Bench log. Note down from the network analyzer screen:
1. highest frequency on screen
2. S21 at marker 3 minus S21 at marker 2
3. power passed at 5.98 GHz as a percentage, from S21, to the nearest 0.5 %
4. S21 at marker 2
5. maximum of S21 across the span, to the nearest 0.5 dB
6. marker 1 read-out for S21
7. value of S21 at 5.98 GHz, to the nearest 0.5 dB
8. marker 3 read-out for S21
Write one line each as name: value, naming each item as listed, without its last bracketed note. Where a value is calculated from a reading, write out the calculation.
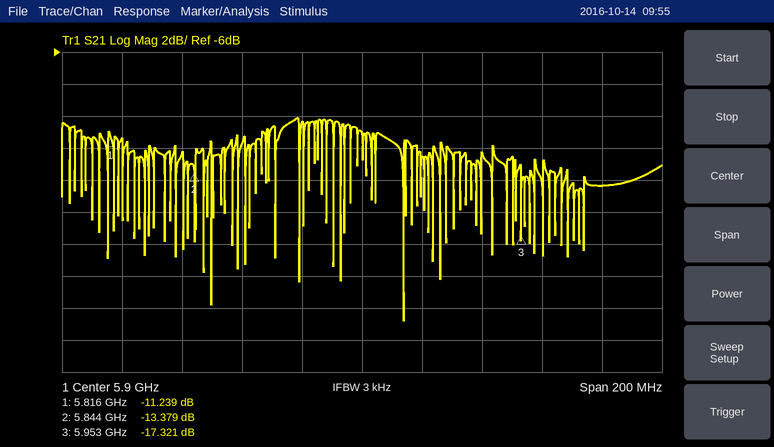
highest frequency on screen: 6 GHz
S21 at marker 3 minus S21 at marker 2: -17.321 − (-13.379) = -3.942 dB
power passed at 5.98 GHz as a percentage, from S21, to the nearest 0.5 %: 10^(-14.5/10) ≈ 3.5 %
S21 at marker 2: -13.379 dB
maximum of S21 across the span, to the nearest 0.5 dB: -10.0 dB
marker 1 read-out for S21: -11.239 dB
value of S21 at 5.98 GHz, to the nearest 0.5 dB: -14.5 dB
marker 3 read-out for S21: -17.321 dB
